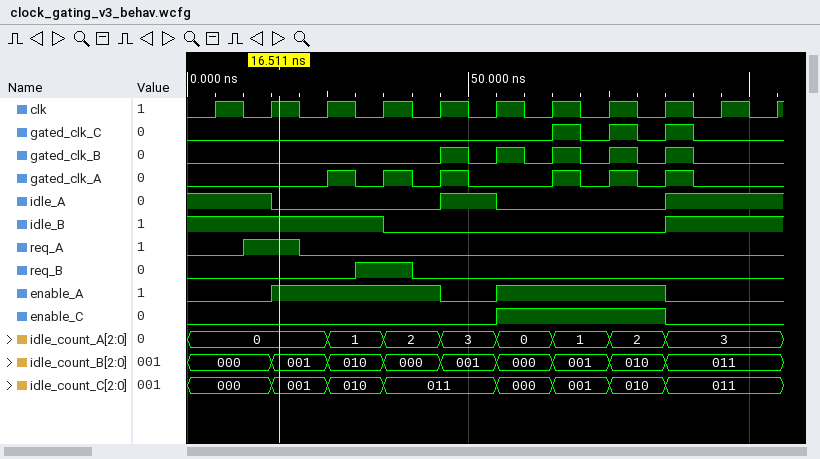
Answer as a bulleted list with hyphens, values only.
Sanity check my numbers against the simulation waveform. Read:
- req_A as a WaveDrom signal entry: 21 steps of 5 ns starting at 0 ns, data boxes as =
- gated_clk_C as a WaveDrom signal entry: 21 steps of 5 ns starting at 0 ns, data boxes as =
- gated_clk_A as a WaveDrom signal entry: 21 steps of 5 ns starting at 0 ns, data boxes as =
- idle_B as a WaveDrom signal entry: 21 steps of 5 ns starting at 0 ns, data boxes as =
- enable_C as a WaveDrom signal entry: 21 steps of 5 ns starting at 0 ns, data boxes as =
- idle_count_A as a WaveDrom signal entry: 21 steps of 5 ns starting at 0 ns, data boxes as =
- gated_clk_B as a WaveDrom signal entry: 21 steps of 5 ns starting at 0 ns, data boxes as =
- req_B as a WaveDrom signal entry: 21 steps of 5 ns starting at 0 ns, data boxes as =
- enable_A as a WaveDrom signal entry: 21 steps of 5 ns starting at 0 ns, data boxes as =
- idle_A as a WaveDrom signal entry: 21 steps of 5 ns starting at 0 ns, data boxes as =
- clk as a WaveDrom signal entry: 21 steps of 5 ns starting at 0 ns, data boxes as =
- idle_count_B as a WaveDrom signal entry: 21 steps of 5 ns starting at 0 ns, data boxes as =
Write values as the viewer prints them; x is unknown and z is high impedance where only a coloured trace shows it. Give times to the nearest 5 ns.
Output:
- {name: 'req_A', wave: '0.1.0................'}
- {name: 'gated_clk_C', wave: '0............101010..'}
- {name: 'gated_clk_A', wave: '0....101010..101010..'}
- {name: 'idle_B', wave: '1......0.........1...'}
- {name: 'enable_C', wave: '0..........1.....0...'}
- {name: 'idle_count_A', wave: '=....=.=.=.=.=.=.=...', data: '0 1 2 3 0 1 2 3'}
- {name: 'gated_clk_B', wave: '0........1010101010..'}
- {name: 'req_B', wave: '0.....1.0............'}
- {name: 'enable_A', wave: '0..1.....0.1.....0...'}
- {name: 'idle_A', wave: '1..0.....1.0.....1...'}
- {name: 'clk', wave: '010101010101010101010'}
- {name: 'idle_count_B', wave: '=..=.=.=.=.=.=.=.=...', data: '000 001 010 000 001 000 001 010 011'}
